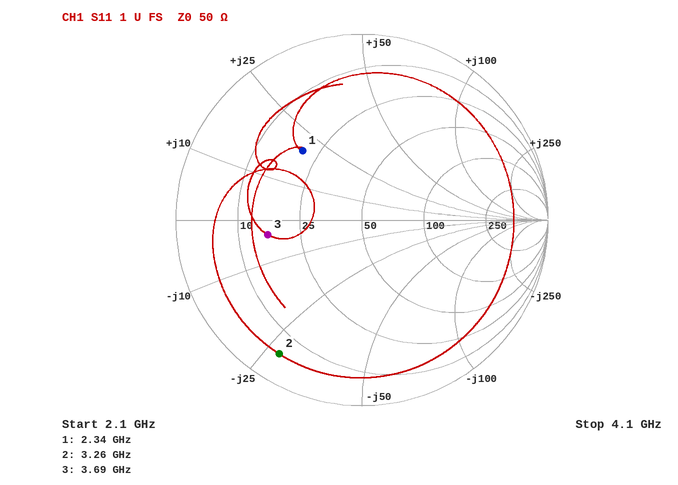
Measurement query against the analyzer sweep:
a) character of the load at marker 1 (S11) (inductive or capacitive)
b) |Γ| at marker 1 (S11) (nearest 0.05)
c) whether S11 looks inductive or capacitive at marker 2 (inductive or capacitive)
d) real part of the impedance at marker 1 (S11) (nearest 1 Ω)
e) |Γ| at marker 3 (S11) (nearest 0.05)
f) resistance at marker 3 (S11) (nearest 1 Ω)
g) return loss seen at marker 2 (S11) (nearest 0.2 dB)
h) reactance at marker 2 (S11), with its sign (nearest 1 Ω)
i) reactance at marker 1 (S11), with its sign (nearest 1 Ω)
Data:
inductive
0.50
capacitive
20 Ω
0.50
16 Ω
1.4 dB
-28 Ω
+20 Ω
